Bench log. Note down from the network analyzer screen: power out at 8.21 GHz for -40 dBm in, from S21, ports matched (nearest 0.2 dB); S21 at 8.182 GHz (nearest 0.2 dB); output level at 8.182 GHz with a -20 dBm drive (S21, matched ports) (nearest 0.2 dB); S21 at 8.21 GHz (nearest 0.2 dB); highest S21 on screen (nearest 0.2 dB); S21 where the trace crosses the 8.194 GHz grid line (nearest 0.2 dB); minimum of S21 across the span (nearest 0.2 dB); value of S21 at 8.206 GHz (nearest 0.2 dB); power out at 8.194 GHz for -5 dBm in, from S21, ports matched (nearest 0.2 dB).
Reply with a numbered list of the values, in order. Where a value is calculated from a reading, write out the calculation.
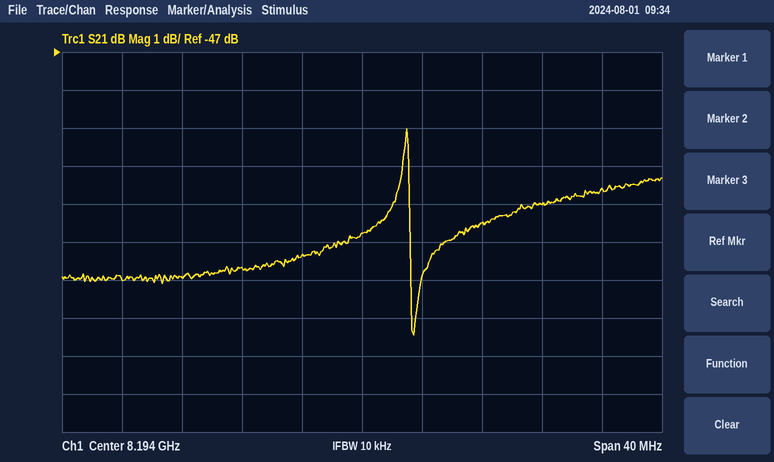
1. -40 dBm + (-50.6 dB) = -90.6 dBm
2. -53.0 dB
3. -20 dBm + (-53.0 dB) = -73.0 dBm
4. -50.6 dB
5. -49.0 dB
6. -51.8 dB
7. -54.4 dB
8. -51.0 dB
9. -5 dBm + (-51.8 dB) = -56.8 dBm
